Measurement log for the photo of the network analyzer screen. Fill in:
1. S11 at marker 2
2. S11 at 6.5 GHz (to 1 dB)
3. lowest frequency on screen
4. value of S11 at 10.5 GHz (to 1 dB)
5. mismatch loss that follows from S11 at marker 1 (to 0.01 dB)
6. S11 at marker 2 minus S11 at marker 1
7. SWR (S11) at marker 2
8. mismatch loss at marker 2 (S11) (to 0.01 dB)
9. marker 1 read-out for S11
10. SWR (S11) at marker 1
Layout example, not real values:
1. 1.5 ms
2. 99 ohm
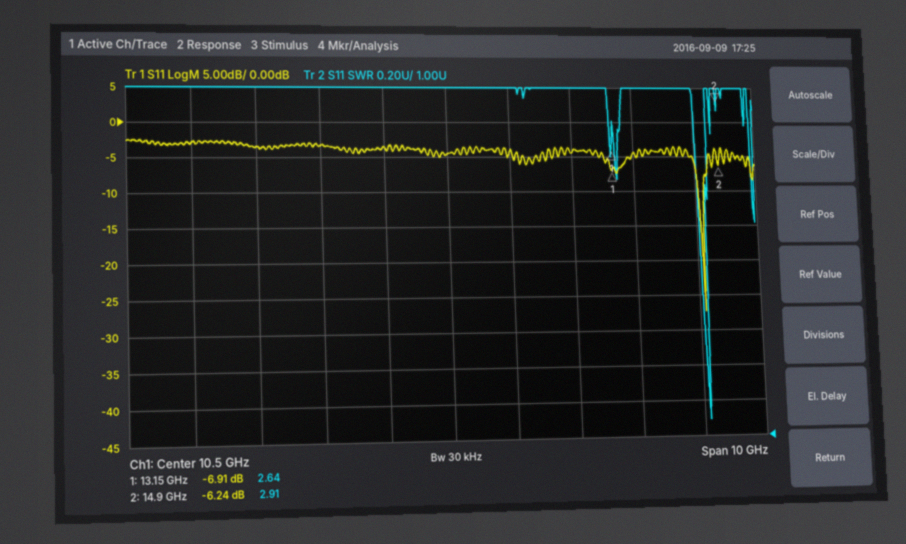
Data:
1. -6.24 dB
2. -3 dB
3. 5.5 GHz
4. -5 dB
5. 0.99 dB
6. 0.67 dB
7. 2.91
8. 1.18 dB
9. -6.91 dB
10. 2.64
